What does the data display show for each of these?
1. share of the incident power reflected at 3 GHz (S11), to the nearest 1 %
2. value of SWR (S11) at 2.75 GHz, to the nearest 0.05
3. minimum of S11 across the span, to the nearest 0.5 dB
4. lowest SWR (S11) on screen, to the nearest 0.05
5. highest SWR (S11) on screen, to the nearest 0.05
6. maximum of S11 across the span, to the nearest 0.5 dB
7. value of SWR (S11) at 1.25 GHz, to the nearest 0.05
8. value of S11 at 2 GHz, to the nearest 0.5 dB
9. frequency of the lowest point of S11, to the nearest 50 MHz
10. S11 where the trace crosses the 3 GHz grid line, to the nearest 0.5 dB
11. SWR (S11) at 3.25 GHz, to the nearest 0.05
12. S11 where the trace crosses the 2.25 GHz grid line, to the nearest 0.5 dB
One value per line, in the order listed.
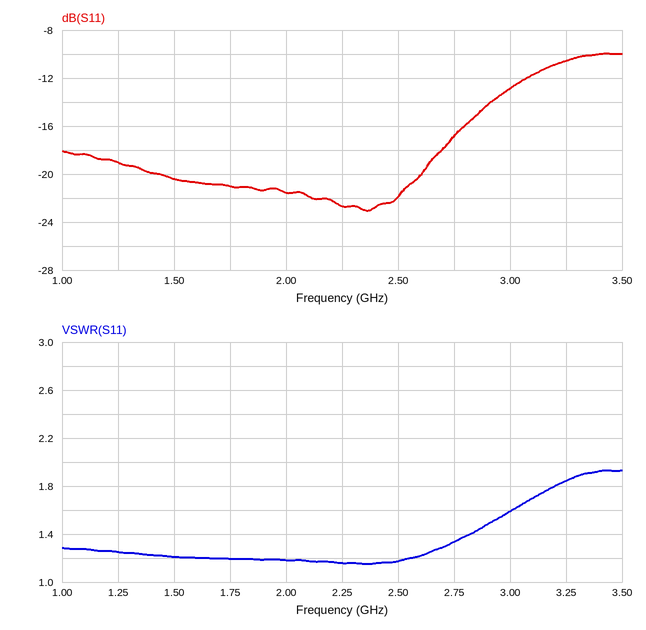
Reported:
5 %
1.35
-23.0 dB
1.15
1.95
-10.0 dB
1.25
-21.5 dB
2.35 GHz
-13.0 dB
1.85
-22.5 dB
